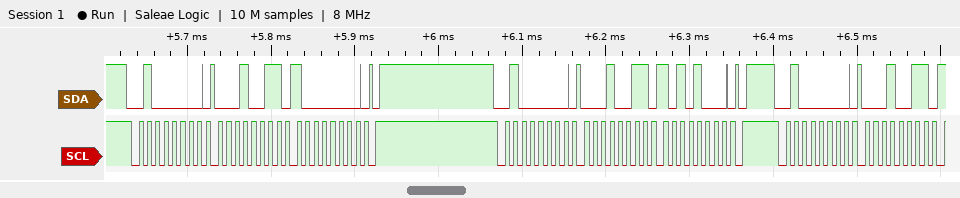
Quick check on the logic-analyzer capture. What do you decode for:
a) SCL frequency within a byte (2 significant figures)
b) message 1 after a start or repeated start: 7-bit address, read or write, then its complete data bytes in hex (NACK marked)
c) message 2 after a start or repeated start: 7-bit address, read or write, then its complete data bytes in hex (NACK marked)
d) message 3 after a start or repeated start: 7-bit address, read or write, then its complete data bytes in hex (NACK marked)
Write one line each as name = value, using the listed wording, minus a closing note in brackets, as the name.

SCL frequency within a byte = 100 kHz
message 1 after a start or repeated start: 7-bit address, read or write, then its complete data bytes in hex = 0x20 write: 13 80
message 2 after a start or repeated start: 7-bit address, read or write, then its complete data bytes in hex = 0x20 write: 13 A8
message 3 after a start or repeated start: 7-bit address, read or write, then its complete data bytes in hex = 0x20 write: 13
